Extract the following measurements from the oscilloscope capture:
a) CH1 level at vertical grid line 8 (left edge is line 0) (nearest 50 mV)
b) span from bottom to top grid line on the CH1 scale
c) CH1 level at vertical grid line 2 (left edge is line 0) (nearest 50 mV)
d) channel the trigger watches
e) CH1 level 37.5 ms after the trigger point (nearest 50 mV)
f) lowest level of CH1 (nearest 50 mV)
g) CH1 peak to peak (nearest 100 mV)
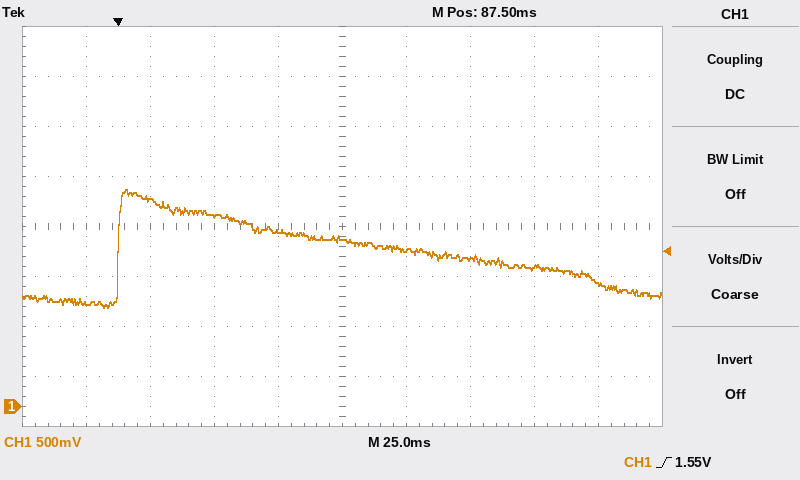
1.40 V
4 V
2.05 V
CH1
1.90 V
1.00 V
1.20 V
